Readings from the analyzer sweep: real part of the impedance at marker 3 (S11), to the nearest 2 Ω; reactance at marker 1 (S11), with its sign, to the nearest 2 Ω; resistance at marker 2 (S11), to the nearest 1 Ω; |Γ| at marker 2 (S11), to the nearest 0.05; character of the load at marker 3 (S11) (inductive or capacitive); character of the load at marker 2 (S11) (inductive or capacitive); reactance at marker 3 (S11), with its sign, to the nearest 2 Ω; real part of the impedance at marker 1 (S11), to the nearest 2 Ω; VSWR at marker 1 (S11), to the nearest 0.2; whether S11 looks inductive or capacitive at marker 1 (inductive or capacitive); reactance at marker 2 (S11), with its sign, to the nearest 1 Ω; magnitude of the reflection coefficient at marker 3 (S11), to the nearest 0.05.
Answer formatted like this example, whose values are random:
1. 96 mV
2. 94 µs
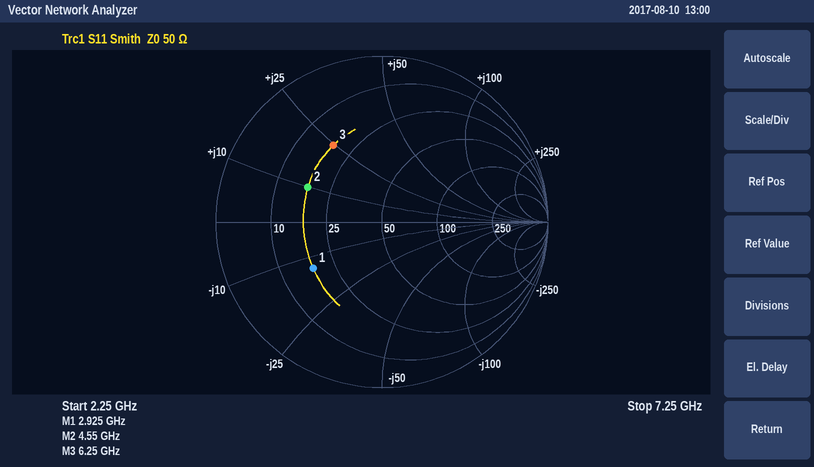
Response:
1. 18 Ω
2. -14 Ω
3. 18 Ω
4. 0.50
5. inductive
6. inductive
7. +24 Ω
8. 18 Ω
9. 3.0
10. capacitive
11. +10 Ω
12. 0.55
